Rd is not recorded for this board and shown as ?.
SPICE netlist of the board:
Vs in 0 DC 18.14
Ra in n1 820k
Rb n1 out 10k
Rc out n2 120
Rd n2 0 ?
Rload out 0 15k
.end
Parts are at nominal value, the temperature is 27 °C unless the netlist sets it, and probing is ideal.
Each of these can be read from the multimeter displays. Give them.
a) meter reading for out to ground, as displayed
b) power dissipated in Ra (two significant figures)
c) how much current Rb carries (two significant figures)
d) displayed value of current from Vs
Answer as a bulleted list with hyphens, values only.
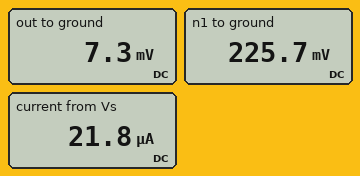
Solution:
- 7.3 mV
- 390 µW
- 22 µA
- 21.8 µA
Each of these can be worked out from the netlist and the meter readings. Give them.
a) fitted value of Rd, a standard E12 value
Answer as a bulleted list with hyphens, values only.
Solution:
- 220 Ω
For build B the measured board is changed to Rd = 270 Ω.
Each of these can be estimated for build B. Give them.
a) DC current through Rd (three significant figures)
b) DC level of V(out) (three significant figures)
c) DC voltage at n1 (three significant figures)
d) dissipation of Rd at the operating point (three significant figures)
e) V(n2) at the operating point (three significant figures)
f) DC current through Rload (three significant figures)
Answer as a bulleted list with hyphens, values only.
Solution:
- 21.3 µA
- 8.30 mV
- 227 mV
- 122 nW
- 5.75 mV
- 554 nA
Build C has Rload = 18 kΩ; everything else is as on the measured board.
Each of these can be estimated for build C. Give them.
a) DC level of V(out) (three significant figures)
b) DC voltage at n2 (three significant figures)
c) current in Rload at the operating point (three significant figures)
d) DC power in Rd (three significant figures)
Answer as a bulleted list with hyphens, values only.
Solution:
- 7.29 mV
- 4.72 mV
- 405 nA
- 101 nW
